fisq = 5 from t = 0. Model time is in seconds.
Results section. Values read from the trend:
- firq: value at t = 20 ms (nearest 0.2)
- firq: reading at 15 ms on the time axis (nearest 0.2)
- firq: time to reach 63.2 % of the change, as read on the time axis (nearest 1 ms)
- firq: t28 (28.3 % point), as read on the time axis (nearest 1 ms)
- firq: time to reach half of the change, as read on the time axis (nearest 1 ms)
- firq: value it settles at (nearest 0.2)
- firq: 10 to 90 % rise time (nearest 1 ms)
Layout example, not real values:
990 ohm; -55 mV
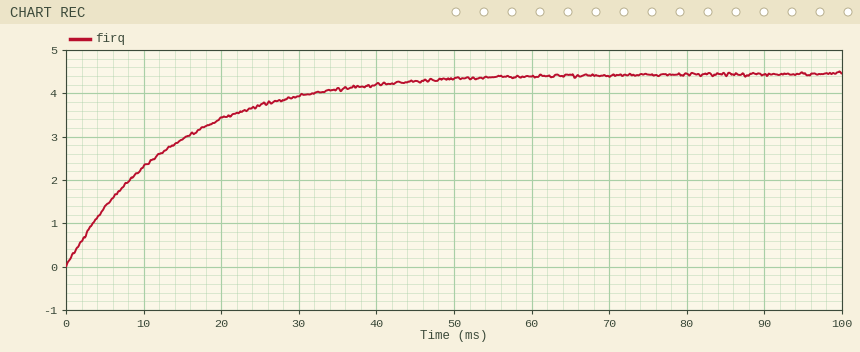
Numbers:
3.4; 3.0; 14 ms; 5 ms; 10 ms; 4.4; 30 ms
